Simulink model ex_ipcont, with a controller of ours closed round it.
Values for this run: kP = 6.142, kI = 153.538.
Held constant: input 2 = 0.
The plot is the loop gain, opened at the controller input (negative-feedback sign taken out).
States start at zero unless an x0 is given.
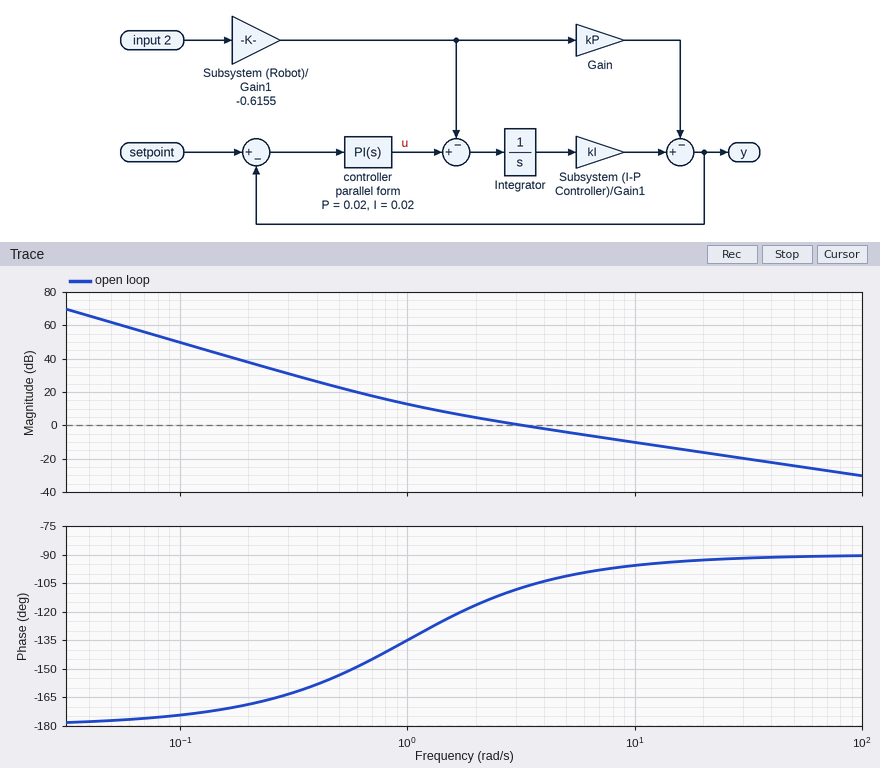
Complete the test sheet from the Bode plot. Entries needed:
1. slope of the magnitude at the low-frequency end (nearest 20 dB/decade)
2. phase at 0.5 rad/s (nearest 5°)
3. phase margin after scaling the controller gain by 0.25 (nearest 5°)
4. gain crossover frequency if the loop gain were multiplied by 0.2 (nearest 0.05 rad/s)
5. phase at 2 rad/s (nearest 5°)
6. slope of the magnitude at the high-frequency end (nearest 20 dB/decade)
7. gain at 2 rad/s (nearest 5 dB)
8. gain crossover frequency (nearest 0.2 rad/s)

-40 dB/decade
-155°
45°
0.90 rad/s
-115°
-20 dB/decade
5 dB
3.2 rad/s
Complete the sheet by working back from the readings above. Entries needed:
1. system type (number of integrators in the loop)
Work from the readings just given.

2
